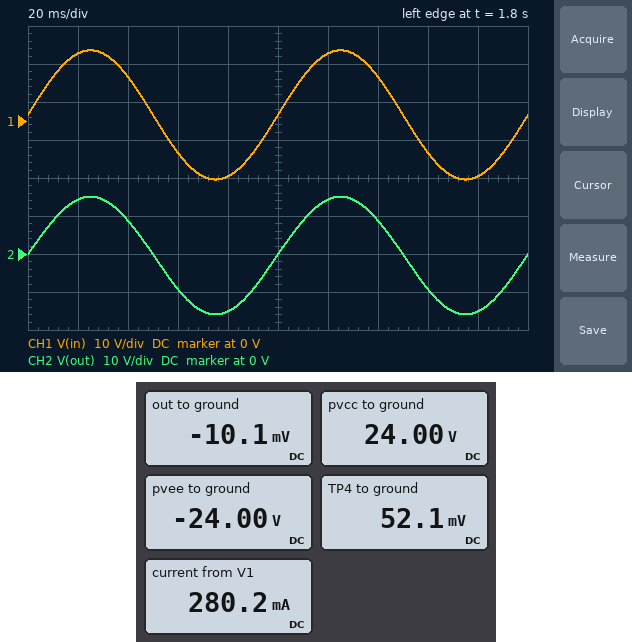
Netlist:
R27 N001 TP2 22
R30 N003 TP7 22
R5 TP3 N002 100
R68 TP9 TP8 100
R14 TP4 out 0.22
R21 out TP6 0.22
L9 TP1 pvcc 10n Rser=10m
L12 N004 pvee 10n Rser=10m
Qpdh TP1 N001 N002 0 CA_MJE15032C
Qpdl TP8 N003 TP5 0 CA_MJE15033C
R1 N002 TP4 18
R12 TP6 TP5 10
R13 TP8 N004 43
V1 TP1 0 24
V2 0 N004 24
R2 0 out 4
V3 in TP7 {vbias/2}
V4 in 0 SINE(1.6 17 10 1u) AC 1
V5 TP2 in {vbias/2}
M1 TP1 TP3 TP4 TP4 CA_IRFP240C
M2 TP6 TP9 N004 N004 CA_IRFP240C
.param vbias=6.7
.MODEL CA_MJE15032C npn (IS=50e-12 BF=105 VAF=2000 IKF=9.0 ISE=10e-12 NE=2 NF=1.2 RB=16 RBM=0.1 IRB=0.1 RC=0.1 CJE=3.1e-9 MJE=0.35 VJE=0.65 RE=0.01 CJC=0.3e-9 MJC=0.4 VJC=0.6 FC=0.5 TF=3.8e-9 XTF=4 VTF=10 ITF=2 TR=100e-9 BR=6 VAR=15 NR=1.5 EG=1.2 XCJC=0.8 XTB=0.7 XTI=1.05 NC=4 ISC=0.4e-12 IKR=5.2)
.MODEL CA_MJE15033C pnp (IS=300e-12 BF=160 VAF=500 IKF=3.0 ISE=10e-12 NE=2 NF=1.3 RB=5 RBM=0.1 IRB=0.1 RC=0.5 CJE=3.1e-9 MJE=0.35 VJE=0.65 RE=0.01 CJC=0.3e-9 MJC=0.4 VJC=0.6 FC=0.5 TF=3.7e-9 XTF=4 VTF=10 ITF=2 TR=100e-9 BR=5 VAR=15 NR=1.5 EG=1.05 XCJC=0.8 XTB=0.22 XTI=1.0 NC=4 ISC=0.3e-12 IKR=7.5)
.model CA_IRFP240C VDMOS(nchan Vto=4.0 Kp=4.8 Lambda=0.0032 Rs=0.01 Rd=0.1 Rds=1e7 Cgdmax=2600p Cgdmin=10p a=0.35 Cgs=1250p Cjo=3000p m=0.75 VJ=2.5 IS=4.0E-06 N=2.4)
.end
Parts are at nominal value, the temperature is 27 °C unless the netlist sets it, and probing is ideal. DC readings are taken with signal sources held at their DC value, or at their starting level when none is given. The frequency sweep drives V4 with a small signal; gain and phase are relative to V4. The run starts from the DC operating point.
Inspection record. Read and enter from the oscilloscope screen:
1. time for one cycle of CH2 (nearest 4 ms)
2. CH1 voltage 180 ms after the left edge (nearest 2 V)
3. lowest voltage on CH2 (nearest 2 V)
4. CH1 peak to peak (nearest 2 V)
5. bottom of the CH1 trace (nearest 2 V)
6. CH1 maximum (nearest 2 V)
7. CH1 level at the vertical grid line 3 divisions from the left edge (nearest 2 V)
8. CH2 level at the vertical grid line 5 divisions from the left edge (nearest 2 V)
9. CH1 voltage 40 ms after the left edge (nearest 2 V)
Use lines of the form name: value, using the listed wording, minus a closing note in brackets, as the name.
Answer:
time for one cycle of CH2: 100 ms
CH1 voltage 180 ms after the left edge: -14 V
lowest voltage on CH2: -16 V
CH1 peak to peak: 34 V
bottom of the CH1 trace: -16 V
CH1 maximum: 18 V
CH1 level at the vertical grid line 3 divisions from the left edge: -8 V
CH2 level at the vertical grid line 5 divisions from the left edge: 0 V
CH1 voltage 40 ms after the left edge: 12 V
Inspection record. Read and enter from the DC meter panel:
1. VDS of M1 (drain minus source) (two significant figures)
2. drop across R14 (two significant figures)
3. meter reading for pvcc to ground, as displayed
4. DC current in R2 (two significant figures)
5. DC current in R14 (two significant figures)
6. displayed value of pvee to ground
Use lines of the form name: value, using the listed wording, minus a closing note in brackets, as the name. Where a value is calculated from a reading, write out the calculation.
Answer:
VDS of M1 (drain minus source): 24 V - 52.1 mV = 24 V
drop across R14: 52.1 mV - (-10.1 mV) = 62 mV
meter reading for pvcc to ground, as displayed: 24.00 V
DC current in R2: (0 V - (-10.1 mV)) / 4 Ω = 2.5 mA
DC current in R14: (52.1 mV - (-10.1 mV)) / 220 mΩ = 280 mA
displayed value of pvee to ground: -24.00 V
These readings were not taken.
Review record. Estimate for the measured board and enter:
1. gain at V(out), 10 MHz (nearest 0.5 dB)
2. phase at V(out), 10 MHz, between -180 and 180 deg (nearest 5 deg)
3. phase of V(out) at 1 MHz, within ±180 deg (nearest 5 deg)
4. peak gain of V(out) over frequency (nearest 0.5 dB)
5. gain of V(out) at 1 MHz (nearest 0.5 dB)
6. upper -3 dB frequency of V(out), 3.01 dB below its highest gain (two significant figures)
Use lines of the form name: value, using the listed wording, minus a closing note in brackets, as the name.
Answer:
gain at V(out), 10 MHz: -4.5 dB
phase at V(out), 10 MHz, between -180 and 180 deg: -110 deg
phase of V(out) at 1 MHz, within ±180 deg: -5 deg
peak gain of V(out) over frequency: 0.5 dB
gain of V(out) at 1 MHz: -0.5 dB
upper -3 dB frequency of V(out), 3.01 dB below its highest gain: 8.8 MHz
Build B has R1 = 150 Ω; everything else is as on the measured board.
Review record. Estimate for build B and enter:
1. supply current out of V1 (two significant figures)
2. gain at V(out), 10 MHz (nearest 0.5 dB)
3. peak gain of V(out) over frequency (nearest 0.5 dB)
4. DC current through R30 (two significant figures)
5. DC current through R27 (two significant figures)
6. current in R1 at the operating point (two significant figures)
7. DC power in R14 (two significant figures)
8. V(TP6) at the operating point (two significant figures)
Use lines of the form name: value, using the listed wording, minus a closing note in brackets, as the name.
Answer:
supply current out of V1: 240 mA
gain at V(out), 10 MHz: -4.5 dB
peak gain of V(out) over frequency: 0 dB
DC current through R30: 640 µA
DC current through R27: 280 µA
current in R1 at the operating point: 29 mA
DC power in R14: 13 mW
V(TP6) at the operating point: -80 mV
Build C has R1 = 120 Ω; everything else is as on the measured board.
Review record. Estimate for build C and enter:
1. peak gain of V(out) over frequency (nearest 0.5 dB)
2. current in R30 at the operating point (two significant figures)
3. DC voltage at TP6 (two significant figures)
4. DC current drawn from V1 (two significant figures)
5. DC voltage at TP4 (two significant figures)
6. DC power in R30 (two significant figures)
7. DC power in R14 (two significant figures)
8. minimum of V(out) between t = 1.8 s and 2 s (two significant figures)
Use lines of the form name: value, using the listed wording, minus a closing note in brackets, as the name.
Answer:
peak gain of V(out) over frequency: 0 dB
current in R30 at the operating point: 640 µA
DC voltage at TP6: -81 mV
DC current drawn from V1: 240 mA
DC voltage at TP4: 26 mV
DC power in R30: 9.1 µW
DC power in R14: 13 mW
minimum of V(out) between t = 1.8 s and 2 s: -16 V
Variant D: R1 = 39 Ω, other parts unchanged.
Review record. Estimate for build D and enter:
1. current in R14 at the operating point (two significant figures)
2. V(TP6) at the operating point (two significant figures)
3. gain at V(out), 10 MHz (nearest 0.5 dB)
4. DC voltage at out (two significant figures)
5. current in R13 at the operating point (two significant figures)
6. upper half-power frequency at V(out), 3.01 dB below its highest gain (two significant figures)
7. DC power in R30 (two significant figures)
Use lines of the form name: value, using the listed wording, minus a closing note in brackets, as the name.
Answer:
current in R14 at the operating point: 240 mA
V(TP6) at the operating point: -81 mV
gain at V(out), 10 MHz: -5.0 dB
DC voltage at out: -27 mV
current in R13 at the operating point: 98 mA
upper half-power frequency at V(out), 3.01 dB below its highest gain: 8.7 MHz
DC power in R30: 9.1 µW
